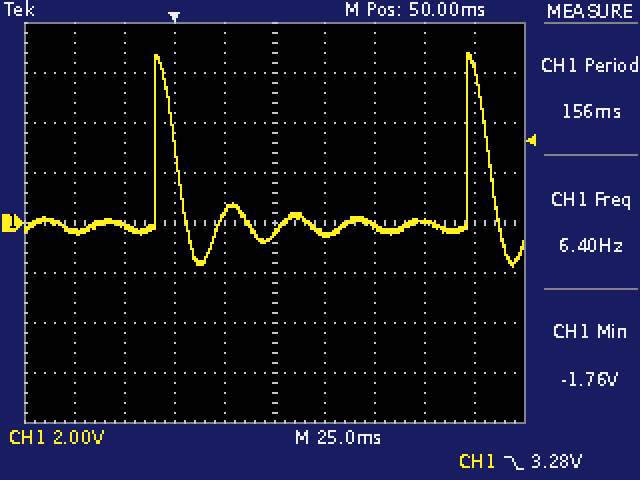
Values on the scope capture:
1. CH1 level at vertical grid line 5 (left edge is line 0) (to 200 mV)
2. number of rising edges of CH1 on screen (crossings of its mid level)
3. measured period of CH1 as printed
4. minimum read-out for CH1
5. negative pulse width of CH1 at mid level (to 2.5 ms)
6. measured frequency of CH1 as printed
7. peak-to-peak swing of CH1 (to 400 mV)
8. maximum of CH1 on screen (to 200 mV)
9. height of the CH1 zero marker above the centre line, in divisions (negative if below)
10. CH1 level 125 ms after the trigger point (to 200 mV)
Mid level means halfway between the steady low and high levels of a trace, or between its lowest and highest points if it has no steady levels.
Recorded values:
-400 mV
2
156 ms
-1.76 V
145.0 ms
6.40 Hz
8.4 V
6.8 V
0.0 div
0.0 V
